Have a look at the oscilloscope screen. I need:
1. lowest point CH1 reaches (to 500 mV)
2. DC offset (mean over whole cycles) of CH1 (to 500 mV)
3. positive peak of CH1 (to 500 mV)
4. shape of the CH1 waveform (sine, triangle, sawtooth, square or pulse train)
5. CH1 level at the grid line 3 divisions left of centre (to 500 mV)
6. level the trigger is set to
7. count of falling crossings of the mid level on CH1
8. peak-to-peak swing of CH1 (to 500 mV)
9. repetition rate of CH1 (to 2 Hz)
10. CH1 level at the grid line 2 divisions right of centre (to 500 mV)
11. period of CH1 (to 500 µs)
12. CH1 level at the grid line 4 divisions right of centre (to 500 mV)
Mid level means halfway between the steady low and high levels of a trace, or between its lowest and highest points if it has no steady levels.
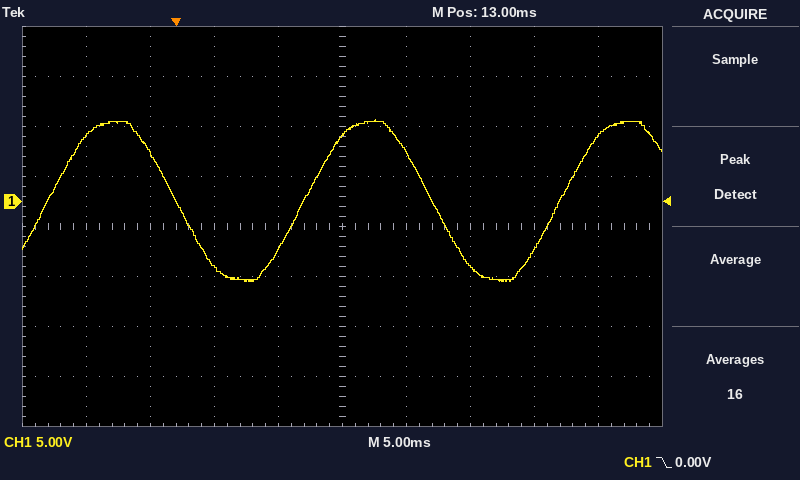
-8.0 V
0.0 V
8.0 V
sine
5.0 V
0.00 V
2
16.0 V
50 Hz
-6.5 V
20.0 ms
6.5 V
